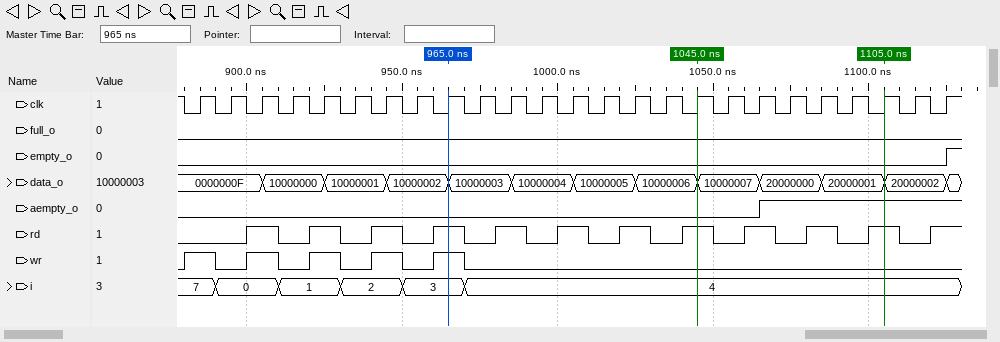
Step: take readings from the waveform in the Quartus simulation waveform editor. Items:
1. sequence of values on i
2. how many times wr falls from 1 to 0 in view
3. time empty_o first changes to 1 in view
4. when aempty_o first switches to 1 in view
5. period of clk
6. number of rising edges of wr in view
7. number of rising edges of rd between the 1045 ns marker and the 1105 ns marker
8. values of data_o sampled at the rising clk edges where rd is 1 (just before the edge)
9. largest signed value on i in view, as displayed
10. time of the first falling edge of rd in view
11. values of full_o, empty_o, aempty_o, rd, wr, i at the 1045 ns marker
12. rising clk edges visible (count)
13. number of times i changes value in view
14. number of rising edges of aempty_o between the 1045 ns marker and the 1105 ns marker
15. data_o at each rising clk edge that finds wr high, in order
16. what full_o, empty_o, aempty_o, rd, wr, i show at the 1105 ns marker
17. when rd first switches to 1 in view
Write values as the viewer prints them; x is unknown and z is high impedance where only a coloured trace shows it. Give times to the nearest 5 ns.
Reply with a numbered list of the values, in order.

1. 7, 0, 1, 2, 3, 4
2. 5
3. 1125 ns
4. 1065 ns
5. 10 ns
6. 5
7. 3
8. 0000000F, 10000000, 10000001, 10000002, 10000003, 10000004, 10000005, 10000006, 10000007, 20000000, 20000001, 20000002
9. 7
10. 910 ns
11. full_o=0, empty_o=0, aempty_o=0, rd=1, wr=0, i=4
12. 25
13. 5
14. 1
15. 0000000F, 0000000F, 10000000, 10000001, 10000002
16. full_o=0, empty_o=0, aempty_o=1, rd=1, wr=0, i=4
17. 900 ns
